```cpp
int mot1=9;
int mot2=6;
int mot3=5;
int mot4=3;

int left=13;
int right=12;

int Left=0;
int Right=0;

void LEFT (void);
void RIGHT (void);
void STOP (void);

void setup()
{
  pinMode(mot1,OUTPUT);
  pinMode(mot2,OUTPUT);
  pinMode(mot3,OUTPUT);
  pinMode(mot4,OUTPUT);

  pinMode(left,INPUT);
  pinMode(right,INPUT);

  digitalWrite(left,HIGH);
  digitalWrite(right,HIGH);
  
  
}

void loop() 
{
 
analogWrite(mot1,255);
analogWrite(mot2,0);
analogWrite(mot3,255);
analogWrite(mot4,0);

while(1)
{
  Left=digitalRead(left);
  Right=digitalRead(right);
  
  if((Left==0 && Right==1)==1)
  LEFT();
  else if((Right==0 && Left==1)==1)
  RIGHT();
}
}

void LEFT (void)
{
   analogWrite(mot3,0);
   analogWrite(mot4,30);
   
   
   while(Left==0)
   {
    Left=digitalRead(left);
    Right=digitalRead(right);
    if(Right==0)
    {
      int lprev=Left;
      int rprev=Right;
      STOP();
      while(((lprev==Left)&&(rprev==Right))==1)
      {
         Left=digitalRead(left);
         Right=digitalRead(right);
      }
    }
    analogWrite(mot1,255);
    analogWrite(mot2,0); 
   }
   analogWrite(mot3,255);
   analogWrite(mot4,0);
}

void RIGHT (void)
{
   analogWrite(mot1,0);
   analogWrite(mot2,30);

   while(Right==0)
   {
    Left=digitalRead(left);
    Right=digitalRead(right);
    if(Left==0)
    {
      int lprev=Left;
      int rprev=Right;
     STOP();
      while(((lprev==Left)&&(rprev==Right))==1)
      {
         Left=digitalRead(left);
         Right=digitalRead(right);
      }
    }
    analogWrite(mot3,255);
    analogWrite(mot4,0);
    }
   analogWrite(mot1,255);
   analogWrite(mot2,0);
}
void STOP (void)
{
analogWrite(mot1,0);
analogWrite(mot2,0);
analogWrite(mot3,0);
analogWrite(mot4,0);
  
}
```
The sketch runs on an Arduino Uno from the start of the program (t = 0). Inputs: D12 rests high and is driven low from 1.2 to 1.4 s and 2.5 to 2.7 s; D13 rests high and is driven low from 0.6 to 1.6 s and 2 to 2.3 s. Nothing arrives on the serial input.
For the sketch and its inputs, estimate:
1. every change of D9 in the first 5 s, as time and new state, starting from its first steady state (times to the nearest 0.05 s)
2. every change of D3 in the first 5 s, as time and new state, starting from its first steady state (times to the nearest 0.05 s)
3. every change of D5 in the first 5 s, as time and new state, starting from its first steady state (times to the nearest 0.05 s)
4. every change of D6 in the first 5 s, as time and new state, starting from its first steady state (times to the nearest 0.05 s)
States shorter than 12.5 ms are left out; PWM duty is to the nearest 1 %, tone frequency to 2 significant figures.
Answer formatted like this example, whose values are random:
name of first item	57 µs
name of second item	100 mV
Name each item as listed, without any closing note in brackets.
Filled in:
every change of D9 in the first 5 s, as time and new state, starting from its first steady state	0 s high; 1.2 s low; 1.4 s high; 2.5 s low; 2.7 s high
every change of D3 in the first 5 s, as time and new state, starting from its first steady state	0 s low; 0.6 s PWM 12 %; 1.2 s low; 2 s PWM 12 %; 2.3 s low
every change of D5 in the first 5 s, as time and new state, starting from its first steady state	0 s high; 0.6 s low; 1.6 s high; 2 s low; 2.3 s high
every change of D6 in the first 5 s, as time and new state, starting from its first steady state	0 s low; 2.5 s PWM 12 %; 2.7 s low
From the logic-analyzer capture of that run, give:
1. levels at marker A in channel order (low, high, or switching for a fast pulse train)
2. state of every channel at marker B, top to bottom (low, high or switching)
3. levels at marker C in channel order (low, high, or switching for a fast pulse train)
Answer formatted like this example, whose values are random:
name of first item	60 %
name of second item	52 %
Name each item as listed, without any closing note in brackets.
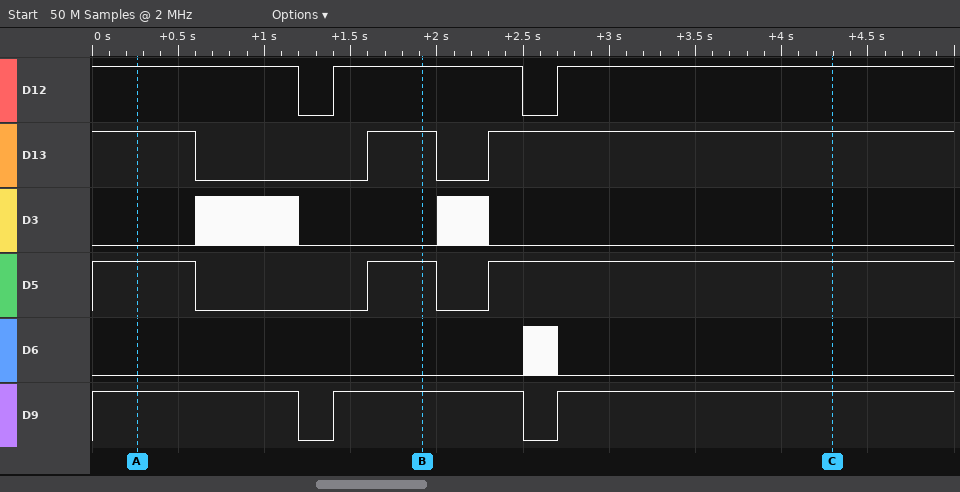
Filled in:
levels at marker A in channel order	D12 high, D13 high, D3 low, D5 high, D6 low, D9 high
state of every channel at marker B, top to bottom	D12 high, D13 high, D3 low, D5 high, D6 low, D9 high
levels at marker C in channel order	D12 high, D13 high, D3 low, D5 high, D6 low, D9 high
